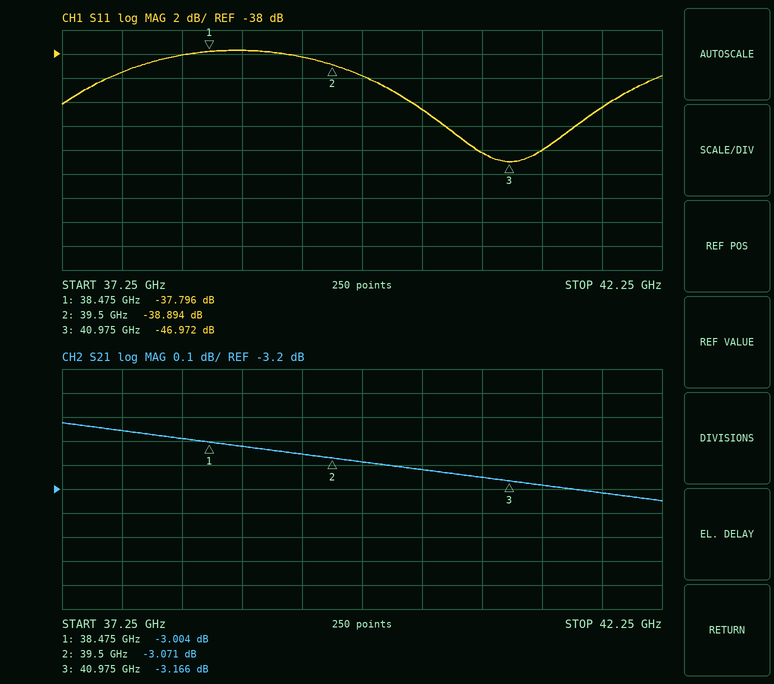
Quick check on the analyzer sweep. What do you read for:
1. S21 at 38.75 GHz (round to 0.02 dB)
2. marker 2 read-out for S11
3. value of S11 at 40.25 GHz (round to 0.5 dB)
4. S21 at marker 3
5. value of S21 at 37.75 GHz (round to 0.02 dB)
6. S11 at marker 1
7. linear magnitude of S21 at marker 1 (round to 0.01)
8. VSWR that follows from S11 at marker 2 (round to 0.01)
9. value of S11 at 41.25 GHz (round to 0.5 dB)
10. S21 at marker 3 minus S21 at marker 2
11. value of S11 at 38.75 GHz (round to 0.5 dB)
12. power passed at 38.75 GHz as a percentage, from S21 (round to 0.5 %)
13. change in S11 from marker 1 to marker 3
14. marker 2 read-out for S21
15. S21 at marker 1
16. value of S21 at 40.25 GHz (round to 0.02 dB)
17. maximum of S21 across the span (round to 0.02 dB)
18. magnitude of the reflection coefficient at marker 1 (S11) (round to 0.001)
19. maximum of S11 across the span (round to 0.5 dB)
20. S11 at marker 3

-3.02 dB
-38.894 dB
-42.5 dB
-3.166 dB
-2.96 dB
-37.796 dB
0.71
1.02
-46.0 dB
-0.095 dB
-37.5 dB
50.0 %
-9.176 dB
-3.071 dB
-3.004 dB
-3.12 dB
-2.92 dB
0.013
-37.5 dB
-46.972 dB
